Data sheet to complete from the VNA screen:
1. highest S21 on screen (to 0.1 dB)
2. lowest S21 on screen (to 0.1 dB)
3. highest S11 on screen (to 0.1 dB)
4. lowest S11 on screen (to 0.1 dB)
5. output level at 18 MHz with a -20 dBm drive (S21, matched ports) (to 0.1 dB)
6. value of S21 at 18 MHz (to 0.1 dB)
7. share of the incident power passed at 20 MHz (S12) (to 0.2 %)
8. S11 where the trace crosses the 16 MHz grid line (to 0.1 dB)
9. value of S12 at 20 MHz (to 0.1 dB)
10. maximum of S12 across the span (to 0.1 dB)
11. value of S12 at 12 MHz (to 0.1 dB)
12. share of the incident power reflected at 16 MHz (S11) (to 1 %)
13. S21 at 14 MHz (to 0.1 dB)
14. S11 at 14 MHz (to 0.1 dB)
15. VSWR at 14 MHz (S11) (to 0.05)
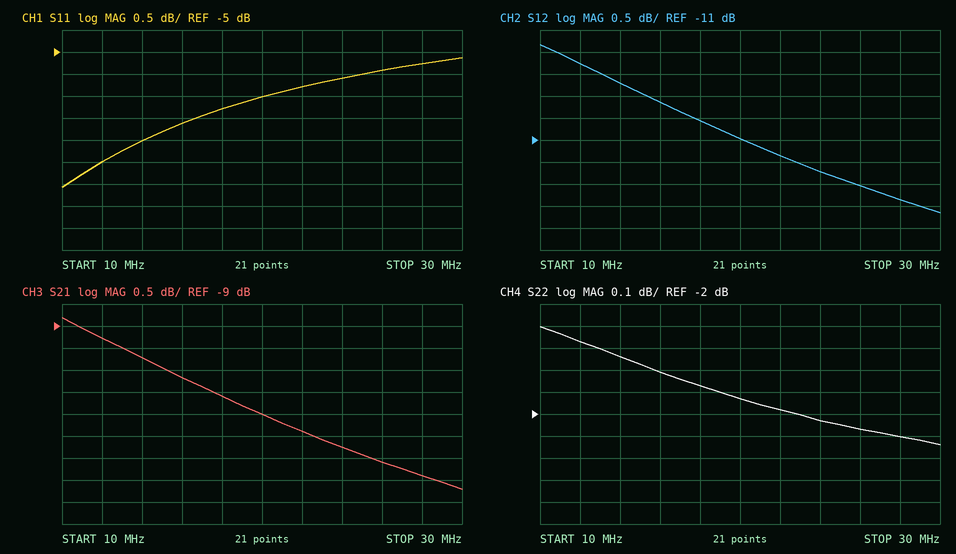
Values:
-8.8 dB
-12.7 dB
-5.1 dB
-8.1 dB
-30.6 dBm
-10.6 dB
8.0 %
-6.6 dB
-11.0 dB
-8.8 dB
-9.3 dB
22 %
-9.7 dB
-7.0 dB
2.60
